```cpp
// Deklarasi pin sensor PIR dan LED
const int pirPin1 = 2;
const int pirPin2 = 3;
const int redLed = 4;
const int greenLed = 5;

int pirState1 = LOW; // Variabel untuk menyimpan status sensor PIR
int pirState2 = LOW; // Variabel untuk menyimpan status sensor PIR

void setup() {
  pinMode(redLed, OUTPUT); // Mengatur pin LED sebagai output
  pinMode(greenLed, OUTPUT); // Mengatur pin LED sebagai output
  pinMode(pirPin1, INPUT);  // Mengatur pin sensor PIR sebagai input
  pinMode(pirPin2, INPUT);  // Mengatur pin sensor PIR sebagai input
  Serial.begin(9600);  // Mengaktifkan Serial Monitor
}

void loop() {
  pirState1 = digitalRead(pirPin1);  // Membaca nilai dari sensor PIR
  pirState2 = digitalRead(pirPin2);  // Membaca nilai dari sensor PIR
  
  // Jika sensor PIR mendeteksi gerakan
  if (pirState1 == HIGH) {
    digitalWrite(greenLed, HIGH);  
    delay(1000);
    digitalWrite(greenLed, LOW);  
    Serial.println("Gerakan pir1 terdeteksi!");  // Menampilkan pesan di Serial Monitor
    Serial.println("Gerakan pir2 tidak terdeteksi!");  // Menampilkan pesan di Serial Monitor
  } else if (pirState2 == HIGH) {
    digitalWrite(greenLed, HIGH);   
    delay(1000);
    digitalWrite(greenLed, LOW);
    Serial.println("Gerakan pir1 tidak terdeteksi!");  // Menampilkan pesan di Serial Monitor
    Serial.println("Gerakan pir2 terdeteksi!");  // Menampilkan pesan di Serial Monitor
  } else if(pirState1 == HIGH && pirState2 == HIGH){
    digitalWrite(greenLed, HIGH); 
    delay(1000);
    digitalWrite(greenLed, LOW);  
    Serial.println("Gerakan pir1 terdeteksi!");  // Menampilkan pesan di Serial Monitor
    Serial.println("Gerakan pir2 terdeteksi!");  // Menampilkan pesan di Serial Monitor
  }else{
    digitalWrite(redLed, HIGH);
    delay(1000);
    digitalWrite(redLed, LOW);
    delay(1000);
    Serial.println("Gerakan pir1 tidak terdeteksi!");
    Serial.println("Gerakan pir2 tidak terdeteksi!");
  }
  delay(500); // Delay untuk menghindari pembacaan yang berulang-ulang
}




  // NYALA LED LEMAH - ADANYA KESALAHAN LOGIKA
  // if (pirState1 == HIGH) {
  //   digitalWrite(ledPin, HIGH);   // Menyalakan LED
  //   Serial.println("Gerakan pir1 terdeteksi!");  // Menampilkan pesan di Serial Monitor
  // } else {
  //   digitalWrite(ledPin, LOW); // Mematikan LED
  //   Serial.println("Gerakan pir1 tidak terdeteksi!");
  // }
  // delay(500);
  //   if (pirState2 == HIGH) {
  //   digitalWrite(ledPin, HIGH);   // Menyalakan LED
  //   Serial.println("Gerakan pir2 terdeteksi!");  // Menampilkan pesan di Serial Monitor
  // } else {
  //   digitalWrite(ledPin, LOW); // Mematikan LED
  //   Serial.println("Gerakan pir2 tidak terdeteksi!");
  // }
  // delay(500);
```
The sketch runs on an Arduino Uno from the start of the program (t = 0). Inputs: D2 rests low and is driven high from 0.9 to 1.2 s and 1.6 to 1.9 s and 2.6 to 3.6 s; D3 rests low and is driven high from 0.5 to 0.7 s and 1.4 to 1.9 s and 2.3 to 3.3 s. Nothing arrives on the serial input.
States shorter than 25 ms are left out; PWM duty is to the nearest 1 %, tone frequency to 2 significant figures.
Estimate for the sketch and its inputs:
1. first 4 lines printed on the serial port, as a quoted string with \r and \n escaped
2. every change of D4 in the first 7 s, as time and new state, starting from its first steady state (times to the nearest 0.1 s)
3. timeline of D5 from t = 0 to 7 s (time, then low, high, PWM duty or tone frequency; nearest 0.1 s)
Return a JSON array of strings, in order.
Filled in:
["\"Gerakan pir1 tidak terdeteksi!\\r\\nGerakan pir2 tidak terdeteksi!\\r\\nGerakan pir1 tidak terdeteksi!\\r\\nGerakan pir2 terdeteksi!\\r\\n\"", "0 s high; 1 s low; 4 s high; 5 s low; 6.5 s high", "0 s low; 2.5 s high; 3.5 s low"]
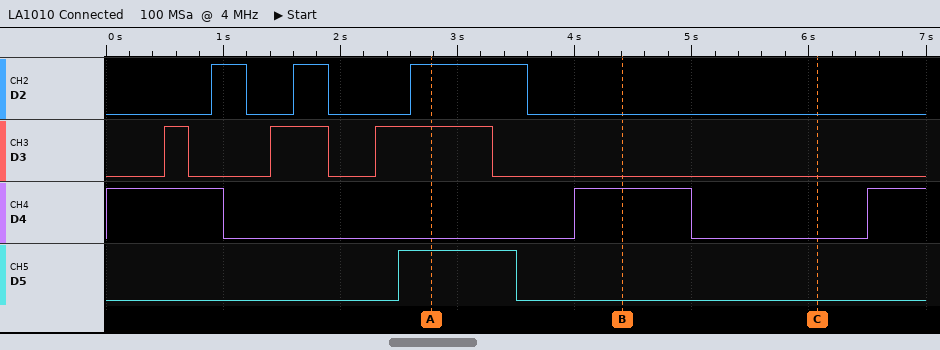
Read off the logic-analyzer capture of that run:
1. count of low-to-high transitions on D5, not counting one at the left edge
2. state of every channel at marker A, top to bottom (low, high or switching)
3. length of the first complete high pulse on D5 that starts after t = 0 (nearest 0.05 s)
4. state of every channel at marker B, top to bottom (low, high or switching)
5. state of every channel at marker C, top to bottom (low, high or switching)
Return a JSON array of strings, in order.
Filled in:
["1", "D2 high, D3 high, D4 low, D5 high", "1.00 s", "D2 low, D3 low, D4 high, D5 low", "D2 low, D3 low, D4 low, D5 low"]
